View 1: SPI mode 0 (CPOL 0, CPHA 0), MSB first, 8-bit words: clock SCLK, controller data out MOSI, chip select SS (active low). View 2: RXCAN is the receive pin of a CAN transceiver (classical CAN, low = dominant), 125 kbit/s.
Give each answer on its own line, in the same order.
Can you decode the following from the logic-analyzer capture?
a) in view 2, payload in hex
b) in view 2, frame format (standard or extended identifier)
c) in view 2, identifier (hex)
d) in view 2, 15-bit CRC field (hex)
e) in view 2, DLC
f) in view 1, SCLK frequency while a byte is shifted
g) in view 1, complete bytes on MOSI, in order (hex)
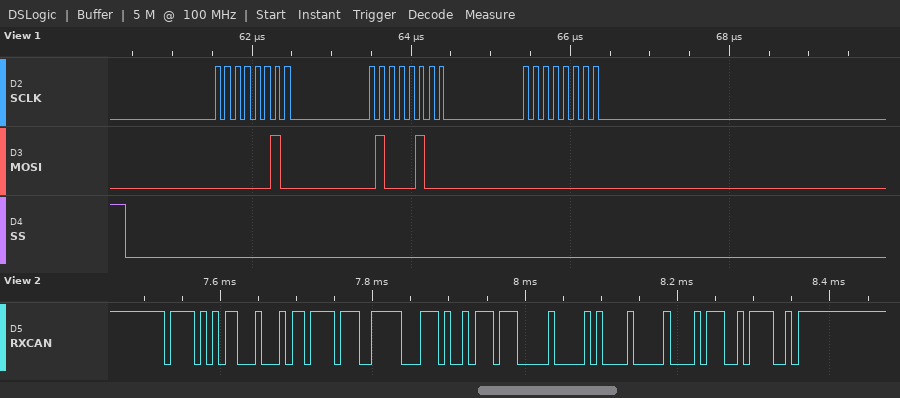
B7 B9 F3 A5 DC 00 42 00
standard
0x7AB
0x5CBC
8
8 MHz
02 44 00
